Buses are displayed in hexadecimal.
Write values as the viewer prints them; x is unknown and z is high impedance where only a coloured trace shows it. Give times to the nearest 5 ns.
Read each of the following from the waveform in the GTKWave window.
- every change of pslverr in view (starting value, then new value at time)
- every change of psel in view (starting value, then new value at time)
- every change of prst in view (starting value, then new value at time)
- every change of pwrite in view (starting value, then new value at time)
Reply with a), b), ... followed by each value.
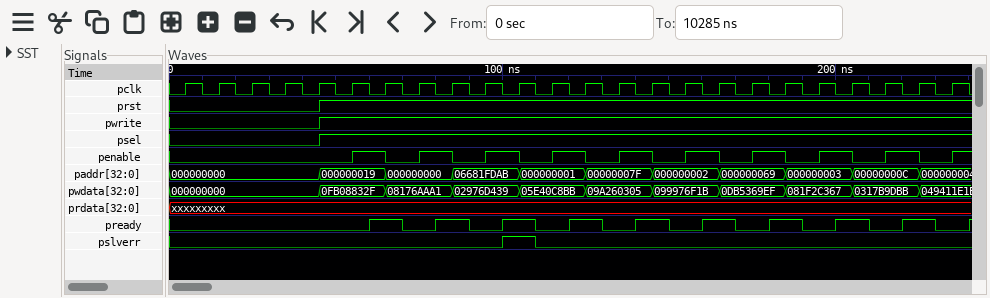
a) 0, 1 at 100 ns, 0 at 110 ns
b) 0, 1 at 45 ns
c) 0, 1 at 45 ns
d) 0, 1 at 45 ns
